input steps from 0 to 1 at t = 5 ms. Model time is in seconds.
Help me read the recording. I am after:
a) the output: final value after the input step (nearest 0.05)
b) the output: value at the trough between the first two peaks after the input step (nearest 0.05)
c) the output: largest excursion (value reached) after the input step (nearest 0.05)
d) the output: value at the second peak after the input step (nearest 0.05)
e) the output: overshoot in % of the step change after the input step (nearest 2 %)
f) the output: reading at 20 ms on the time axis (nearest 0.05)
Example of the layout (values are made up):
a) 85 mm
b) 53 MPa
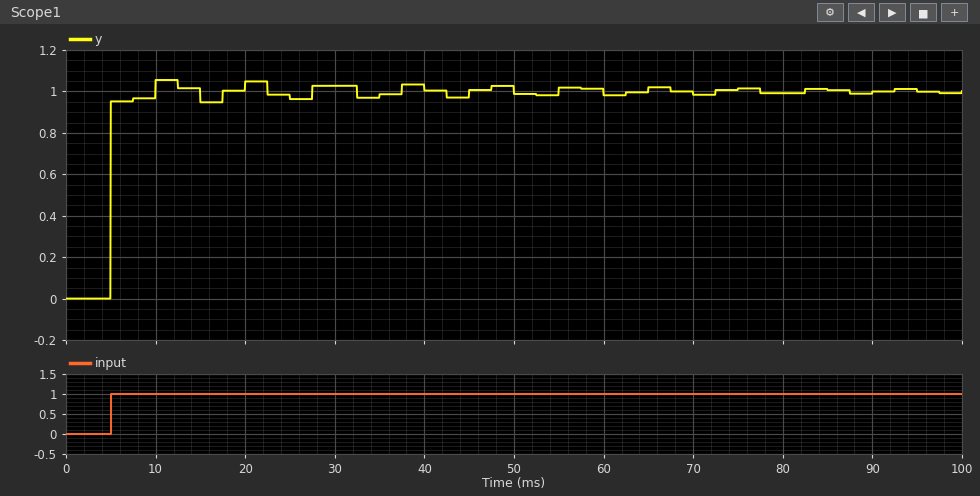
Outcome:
a) 1.00
b) 0.95
c) 1.05
d) 1.05
e) 6 %
f) 1.05
